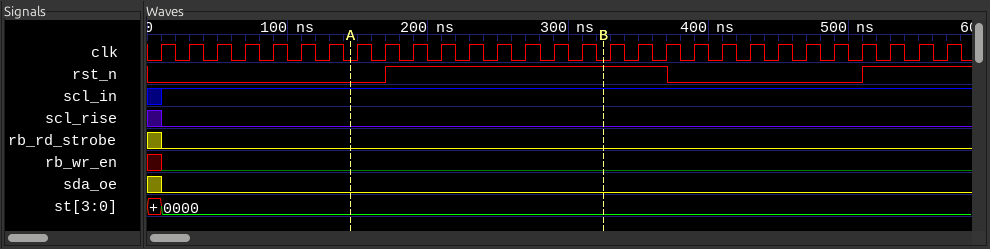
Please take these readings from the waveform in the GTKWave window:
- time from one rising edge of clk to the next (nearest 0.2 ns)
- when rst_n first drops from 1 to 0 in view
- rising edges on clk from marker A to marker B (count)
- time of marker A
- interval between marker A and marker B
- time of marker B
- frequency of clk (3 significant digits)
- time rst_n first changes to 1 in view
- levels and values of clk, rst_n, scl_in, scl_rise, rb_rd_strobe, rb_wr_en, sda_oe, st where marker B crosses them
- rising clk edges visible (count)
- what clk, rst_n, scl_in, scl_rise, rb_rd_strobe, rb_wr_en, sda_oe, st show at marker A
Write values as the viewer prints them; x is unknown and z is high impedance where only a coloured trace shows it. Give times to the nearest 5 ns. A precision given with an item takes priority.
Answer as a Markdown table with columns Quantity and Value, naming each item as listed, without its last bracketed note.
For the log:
| Quantity | Value |
|---|---|
| time from one rising edge of clk to the next | 20 ns |
| when rst_n first drops from 1 to 0 in view | 370 ns |
| rising edges on clk from marker A to marker B | 9 |
| time of marker A | 145 ns |
| interval between marker A and marker B | 180 ns |
| time of marker B | 325 ns |
| frequency of clk | 50.0 MHz |
| time rst_n first changes to 1 in view | 170 ns |
| levels and values of clk, rst_n, scl_in, scl_rise, rb_rd_strobe, rb_wr_en, sda_oe, st where marker B crosses them | clk=0, rst_n=1, scl_in=1, scl_rise=0, rb_rd_strobe=0, rb_wr_en=0, sda_oe=0, st=0000 |
| rising clk edges visible | 29 |
| what clk, rst_n, scl_in, scl_rise, rb_rd_strobe, rb_wr_en, sda_oe, st show at marker A | clk=0, rst_n=0, scl_in=1, scl_rise=0, rb_rd_strobe=0, rb_wr_en=0, sda_oe=0, st=0000 |
